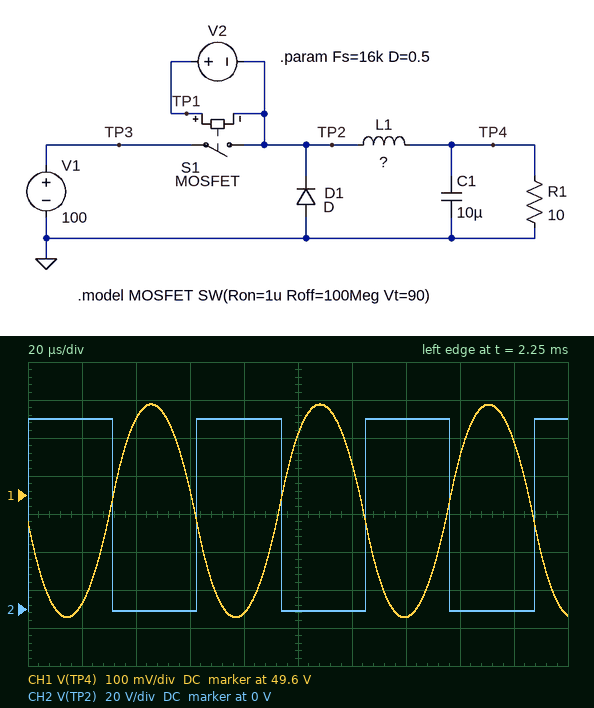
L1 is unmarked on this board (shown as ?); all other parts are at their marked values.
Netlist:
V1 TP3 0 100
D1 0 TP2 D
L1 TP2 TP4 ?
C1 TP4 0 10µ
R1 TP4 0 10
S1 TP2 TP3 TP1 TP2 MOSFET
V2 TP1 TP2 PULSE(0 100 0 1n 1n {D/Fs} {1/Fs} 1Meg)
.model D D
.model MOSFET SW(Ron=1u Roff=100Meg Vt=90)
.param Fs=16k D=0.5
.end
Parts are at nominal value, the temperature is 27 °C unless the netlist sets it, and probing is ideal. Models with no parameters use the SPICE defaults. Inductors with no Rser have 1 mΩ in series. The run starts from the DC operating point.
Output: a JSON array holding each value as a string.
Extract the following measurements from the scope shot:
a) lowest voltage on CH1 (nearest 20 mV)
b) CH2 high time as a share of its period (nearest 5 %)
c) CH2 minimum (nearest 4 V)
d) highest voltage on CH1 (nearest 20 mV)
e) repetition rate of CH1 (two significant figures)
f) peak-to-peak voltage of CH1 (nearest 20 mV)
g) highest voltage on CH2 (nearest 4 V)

["49.28 V", "50 %", "0 V", "49.84 V", "16 kHz", "560 mV", "100 V"]
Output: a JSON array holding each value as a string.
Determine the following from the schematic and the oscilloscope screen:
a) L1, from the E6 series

["2.2 mH"]
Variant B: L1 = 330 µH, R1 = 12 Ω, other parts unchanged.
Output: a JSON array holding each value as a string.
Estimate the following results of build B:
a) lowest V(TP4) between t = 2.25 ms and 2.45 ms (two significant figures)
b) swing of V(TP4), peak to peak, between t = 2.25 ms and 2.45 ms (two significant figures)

["48 V", "3.8 V"]
